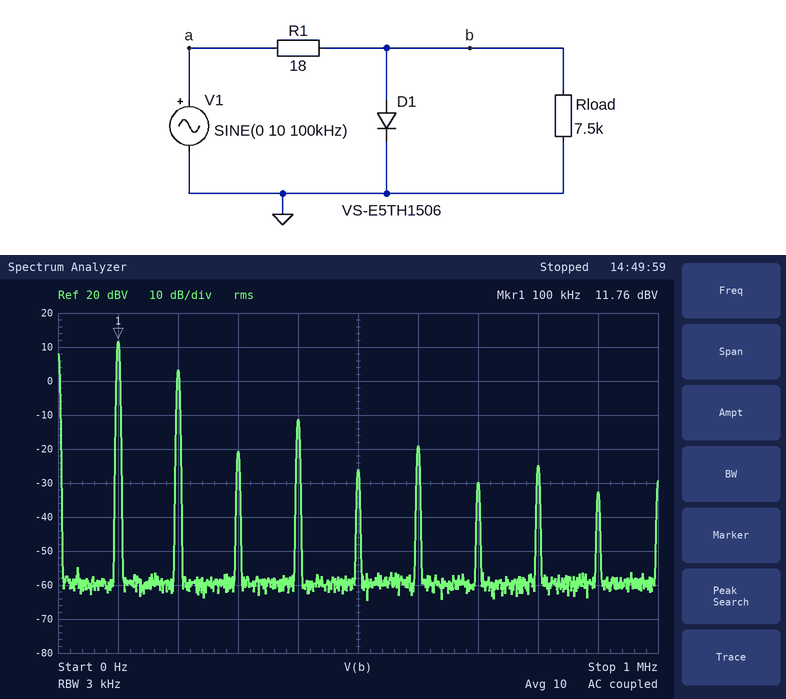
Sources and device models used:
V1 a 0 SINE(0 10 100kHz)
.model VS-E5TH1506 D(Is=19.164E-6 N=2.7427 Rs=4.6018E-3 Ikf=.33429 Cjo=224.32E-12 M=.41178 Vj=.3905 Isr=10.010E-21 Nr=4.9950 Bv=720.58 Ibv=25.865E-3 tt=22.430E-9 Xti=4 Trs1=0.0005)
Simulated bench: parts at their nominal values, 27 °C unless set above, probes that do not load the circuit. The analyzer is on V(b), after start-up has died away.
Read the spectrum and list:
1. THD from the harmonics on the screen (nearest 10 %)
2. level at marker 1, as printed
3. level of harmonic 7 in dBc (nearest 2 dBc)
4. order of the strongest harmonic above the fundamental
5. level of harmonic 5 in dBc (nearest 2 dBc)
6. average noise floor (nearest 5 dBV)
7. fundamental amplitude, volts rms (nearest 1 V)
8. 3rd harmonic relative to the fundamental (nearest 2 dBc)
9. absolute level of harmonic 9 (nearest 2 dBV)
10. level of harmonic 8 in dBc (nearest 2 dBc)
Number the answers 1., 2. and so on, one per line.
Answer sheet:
1. 40 %
2. 11.76 dBV
3. -42 dBc
4. 2
5. -38 dBc
6. -60 dBV
7. 4 V
8. -32 dBc
9. -32 dBV
10. -36 dBc
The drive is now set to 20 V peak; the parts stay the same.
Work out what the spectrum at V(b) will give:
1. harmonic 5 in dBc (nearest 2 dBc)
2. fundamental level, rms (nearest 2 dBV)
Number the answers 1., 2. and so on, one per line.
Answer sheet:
1. -42 dBc
2. 18 dBV
